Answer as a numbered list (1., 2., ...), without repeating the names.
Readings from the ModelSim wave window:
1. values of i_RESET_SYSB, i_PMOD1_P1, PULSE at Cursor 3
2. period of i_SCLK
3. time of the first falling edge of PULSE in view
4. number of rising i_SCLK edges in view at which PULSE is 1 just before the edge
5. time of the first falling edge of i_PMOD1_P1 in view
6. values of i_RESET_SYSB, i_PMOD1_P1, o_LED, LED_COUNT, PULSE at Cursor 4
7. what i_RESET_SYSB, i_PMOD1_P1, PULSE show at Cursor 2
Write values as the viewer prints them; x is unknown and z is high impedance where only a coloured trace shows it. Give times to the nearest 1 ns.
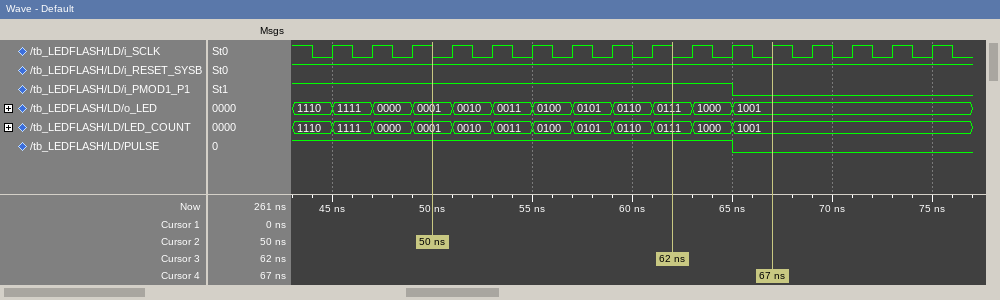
1. i_RESET_SYSB=1, i_PMOD1_P1=1, PULSE=1
2. 2 ns
3. 65 ns
4. 11
5. 65 ns
6. i_RESET_SYSB=1, i_PMOD1_P1=0, o_LED=1001, LED_COUNT=1001, PULSE=0
7. i_RESET_SYSB=1, i_PMOD1_P1=1, PULSE=1
